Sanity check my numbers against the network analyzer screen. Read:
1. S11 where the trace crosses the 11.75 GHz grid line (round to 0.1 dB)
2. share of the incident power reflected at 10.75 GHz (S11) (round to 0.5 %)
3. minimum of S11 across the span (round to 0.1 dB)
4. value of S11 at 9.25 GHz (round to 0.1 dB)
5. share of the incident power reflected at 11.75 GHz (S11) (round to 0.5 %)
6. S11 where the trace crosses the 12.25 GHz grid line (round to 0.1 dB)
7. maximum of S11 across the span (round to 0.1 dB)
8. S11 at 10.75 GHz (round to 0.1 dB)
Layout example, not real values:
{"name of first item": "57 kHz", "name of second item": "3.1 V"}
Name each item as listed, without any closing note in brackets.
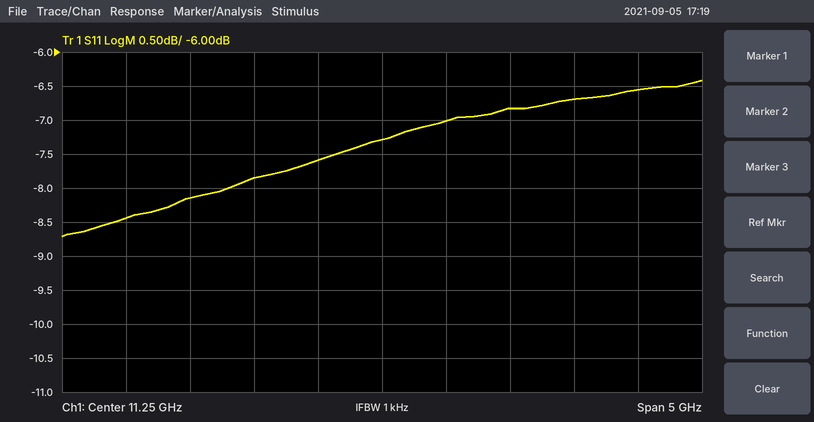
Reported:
{"S11 where the trace crosses the 11.75 GHz grid line": "-7.0 dB", "share of the incident power reflected at 10.75 GHz (S11)": "17.5 %", "minimum of S11 across the span": "-8.7 dB", "value of S11 at 9.25 GHz": "-8.4 dB", "share of the incident power reflected at 11.75 GHz (S11)": "20.0 %", "S11 where the trace crosses the 12.25 GHz grid line": "-6.8 dB", "maximum of S11 across the span": "-6.4 dB", "S11 at 10.75 GHz": "-7.6 dB"}
